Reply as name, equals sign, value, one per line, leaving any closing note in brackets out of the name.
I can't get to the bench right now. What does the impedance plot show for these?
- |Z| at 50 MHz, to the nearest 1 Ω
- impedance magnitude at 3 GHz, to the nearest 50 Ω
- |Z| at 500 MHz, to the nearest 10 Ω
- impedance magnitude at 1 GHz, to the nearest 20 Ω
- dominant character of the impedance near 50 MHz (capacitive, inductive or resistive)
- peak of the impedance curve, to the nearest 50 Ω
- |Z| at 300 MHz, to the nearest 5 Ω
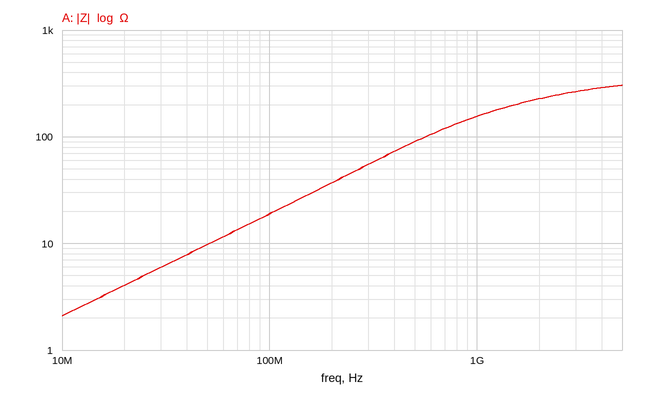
|Z| at 50 MHz, to the nearest 1 Ω = 10 Ω
impedance magnitude at 3 GHz, to the nearest 50 Ω = 250 Ω
|Z| at 500 MHz, to the nearest 10 Ω = 90 Ω
impedance magnitude at 1 GHz, to the nearest 20 Ω = 160 Ω
dominant character of the impedance near 50 MHz = inductive
peak of the impedance curve, to the nearest 50 Ω = 300 Ω
|Z| at 300 MHz, to the nearest 5 Ω = 55 Ω
